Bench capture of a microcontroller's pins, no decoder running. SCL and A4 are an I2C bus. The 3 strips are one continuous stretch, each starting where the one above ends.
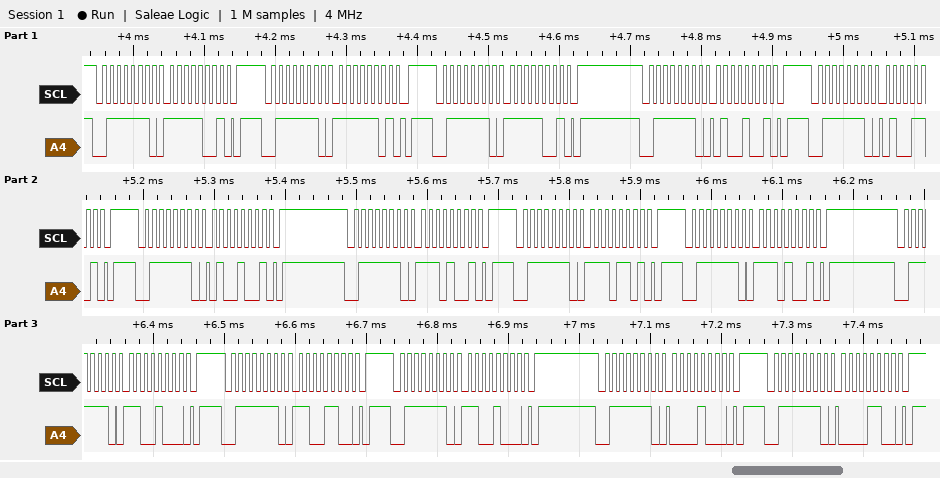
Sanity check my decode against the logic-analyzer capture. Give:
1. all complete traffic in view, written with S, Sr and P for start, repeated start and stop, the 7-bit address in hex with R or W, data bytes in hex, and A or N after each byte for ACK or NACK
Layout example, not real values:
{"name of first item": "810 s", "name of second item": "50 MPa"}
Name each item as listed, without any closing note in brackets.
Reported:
{"all complete traffic in view, written with S, Sr and P for start, repeated start and stop, the 7-bit address in hex with R or W, data bytes in hex, and A or N after each byte for ACK or NACK": "S 3FW A F9 A P S 3FW A FD A P S 3FW A F9 A P S 3FW A 49 A P S 3FW A 4D A P S 3FW A 49 A P S 3FW A E9 A P S 3FW A ED A P S 3FW A E9 A P S 3FW A C8 A P S 3FW A CC A P S 3FW A C8 A P S 3FW A 08 A P S 3FW A 0C A P"}
